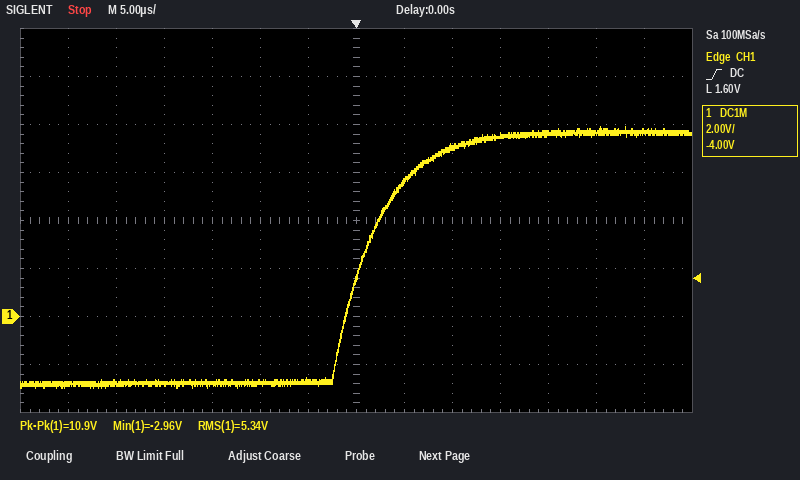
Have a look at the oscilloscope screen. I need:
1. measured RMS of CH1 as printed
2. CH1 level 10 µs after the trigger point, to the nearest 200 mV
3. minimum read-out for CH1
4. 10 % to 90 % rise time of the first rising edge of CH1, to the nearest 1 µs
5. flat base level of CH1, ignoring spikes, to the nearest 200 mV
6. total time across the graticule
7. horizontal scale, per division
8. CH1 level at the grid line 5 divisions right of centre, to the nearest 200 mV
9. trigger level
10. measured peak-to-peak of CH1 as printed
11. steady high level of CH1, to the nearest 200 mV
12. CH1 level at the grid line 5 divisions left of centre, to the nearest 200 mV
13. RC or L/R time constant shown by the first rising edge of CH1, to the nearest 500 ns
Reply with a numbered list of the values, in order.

1. 5.34 V
2. 7.0 V
3. -2.96 V
4. 10 µs
5. -2.8 V
6. 70 µs
7. 5 µs
8. 7.6 V
9. 1.60 V
10. 10.9 V
11. 7.6 V
12. -2.8 V
13. 4.5 µs
